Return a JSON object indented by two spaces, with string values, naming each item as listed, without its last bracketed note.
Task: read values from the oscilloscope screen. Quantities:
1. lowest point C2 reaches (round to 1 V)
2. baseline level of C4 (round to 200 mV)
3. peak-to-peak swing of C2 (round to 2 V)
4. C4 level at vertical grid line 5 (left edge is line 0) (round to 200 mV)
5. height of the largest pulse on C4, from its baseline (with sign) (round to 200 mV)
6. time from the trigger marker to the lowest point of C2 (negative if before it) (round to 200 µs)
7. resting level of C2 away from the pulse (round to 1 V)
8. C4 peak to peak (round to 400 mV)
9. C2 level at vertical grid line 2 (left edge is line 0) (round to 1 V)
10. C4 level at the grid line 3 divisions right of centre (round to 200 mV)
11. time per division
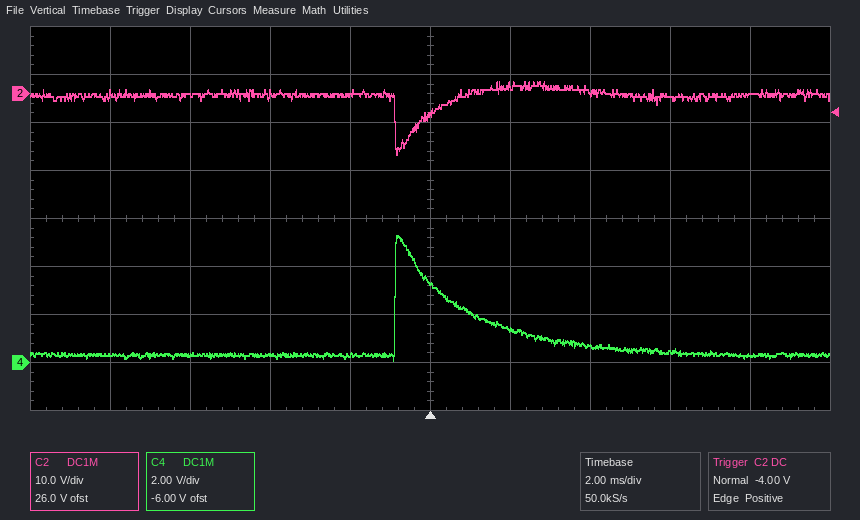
{
  "lowest point C2 reaches": "-13 V",
  "baseline level of C4": "400 mV",
  "peak-to-peak swing of C2": "16 V",
  "C4 level at vertical grid line 5 (left edge is line 0)": "3.4 V",
  "height of the largest pulse on C4, from its baseline (with sign)": "+5.0 V",
  "time from the trigger marker to the lowest point of C2 (negative if before it)": "-800 µs",
  "resting level of C2 away from the pulse": "0 V",
  "C4 peak to peak": "5.2 V",
  "C2 level at vertical grid line 2 (left edge is line 0)": "0 V",
  "C4 level at the grid line 3 divisions right of centre": "400 mV",
  "time per division": "2 ms"
}
